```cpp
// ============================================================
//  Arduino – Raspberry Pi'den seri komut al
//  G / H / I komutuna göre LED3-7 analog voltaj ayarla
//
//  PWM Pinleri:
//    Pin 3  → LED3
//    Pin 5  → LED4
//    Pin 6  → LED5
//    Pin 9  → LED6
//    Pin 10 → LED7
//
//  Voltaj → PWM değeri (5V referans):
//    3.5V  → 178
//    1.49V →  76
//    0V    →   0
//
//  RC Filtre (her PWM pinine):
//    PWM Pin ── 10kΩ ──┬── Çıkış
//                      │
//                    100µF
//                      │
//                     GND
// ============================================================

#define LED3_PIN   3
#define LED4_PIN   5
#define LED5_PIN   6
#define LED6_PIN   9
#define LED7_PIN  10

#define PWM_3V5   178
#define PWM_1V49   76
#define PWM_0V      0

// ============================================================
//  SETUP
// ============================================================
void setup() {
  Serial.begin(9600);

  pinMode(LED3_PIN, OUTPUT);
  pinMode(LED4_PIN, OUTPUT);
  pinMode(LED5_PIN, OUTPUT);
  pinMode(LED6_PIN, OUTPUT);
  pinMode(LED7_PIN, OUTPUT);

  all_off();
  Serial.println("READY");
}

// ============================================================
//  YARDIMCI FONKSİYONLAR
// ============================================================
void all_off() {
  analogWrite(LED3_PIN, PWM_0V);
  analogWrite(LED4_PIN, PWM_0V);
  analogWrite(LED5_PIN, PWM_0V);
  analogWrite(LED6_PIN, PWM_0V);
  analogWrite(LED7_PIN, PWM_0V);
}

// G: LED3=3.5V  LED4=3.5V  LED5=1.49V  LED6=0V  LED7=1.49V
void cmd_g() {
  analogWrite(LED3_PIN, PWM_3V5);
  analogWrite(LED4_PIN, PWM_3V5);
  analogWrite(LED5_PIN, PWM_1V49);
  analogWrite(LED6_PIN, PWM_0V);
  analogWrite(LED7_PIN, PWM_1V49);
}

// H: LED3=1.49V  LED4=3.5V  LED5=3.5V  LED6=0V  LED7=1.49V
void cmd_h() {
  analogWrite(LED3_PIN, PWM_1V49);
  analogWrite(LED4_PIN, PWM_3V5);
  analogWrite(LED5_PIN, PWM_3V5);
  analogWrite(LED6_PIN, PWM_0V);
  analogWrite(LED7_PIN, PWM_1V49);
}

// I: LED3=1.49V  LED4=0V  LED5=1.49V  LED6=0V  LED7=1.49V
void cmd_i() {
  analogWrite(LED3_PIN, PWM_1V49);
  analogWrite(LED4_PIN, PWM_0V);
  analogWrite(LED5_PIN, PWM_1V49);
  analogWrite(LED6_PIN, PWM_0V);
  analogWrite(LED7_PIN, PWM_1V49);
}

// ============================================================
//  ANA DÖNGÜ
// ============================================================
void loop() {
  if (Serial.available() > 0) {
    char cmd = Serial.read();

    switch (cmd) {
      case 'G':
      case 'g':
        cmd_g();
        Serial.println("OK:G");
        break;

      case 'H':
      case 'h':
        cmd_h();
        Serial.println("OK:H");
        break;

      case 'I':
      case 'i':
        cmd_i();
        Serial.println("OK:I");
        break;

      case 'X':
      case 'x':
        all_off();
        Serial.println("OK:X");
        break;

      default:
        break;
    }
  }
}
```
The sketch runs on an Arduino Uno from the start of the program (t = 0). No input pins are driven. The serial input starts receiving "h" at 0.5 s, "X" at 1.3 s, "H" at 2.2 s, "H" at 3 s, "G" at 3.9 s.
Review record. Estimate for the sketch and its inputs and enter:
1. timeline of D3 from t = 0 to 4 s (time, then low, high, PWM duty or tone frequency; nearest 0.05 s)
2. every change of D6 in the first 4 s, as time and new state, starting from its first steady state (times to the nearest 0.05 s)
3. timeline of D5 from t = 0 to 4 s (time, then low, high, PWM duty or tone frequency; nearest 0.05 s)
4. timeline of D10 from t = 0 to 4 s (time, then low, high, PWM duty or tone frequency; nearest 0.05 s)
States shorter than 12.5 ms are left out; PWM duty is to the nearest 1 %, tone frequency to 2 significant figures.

0 s low; 0.5 s PWM 30 %; 1.3 s low; 2.2 s PWM 30 %; 3.9 s PWM 70 %
0 s low; 0.5 s PWM 70 %; 1.3 s low; 2.2 s PWM 70 %; 3.9 s PWM 30 %
0 s low; 0.5 s PWM 70 %; 1.3 s low; 2.2 s PWM 70 %
0 s low; 0.5 s PWM 30 %; 1.3 s low; 2.2 s PWM 30 %
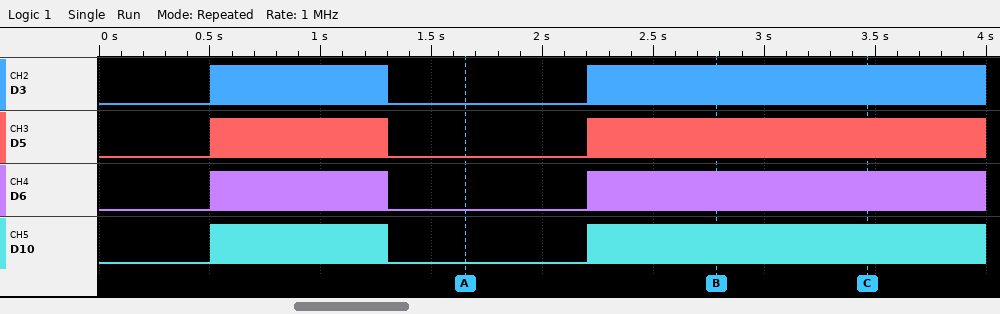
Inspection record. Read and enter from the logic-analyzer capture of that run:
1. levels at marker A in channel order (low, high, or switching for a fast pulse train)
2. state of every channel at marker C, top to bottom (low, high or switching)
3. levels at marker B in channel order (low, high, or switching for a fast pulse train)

D3 low, D5 low, D6 low, D10 low
D3 switching, D5 switching, D6 switching, D10 switching
D3 switching, D5 switching, D6 switching, D10 switching
